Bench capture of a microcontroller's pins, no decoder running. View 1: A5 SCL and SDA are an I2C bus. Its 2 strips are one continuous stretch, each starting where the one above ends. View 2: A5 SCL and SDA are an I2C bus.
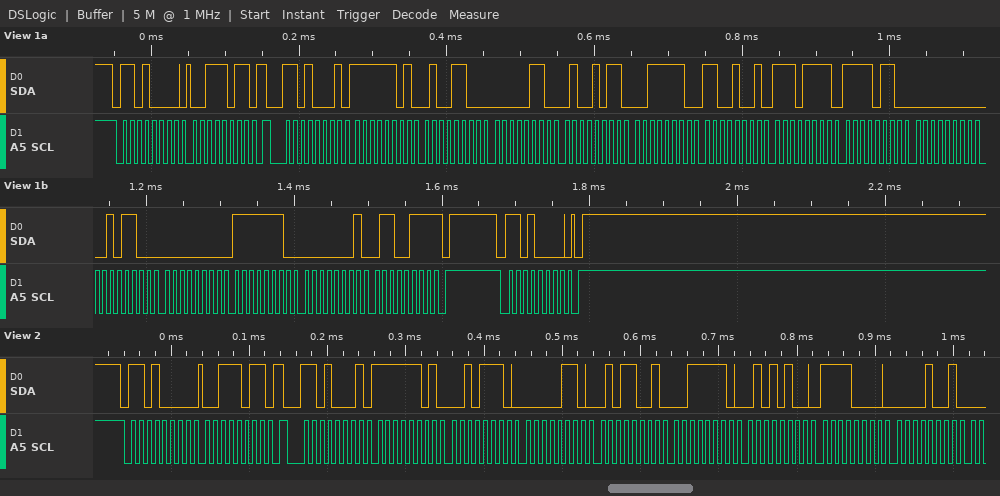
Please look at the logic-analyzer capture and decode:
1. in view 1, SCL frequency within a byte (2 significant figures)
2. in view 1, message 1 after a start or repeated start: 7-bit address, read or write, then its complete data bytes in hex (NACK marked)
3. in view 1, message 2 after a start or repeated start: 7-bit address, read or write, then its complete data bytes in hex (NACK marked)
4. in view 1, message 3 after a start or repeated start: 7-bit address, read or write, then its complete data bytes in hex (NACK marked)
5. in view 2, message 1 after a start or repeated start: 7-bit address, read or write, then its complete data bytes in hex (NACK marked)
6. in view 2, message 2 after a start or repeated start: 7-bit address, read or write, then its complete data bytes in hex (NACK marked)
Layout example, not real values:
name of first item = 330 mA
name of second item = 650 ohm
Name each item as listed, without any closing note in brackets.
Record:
in view 1, SCL frequency within a byte = 100 kHz
in view 1, message 1 after a start or repeated start: 7-bit address, read or write, then its complete data bytes in hex = 0x68 write: 3B
in view 1, message 2 after a start or repeated start: 7-bit address, read or write, then its complete data bytes in hex = 0x68 read: FD 4C 06 4B 3E C9 EF F6 00 2C 00 FE 01 67 NACK
in view 1, message 3 after a start or repeated start: 7-bit address, read or write, then its complete data bytes in hex = 0x68 write
in view 2, message 1 after a start or repeated start: 7-bit address, read or write, then its complete data bytes in hex = 0x68 write: 3B
in view 2, message 2 after a start or repeated start: 7-bit address, read or write, then its complete data bytes in hex = 0x68 read: FD 2E 06 59 3E 54 F0 09
